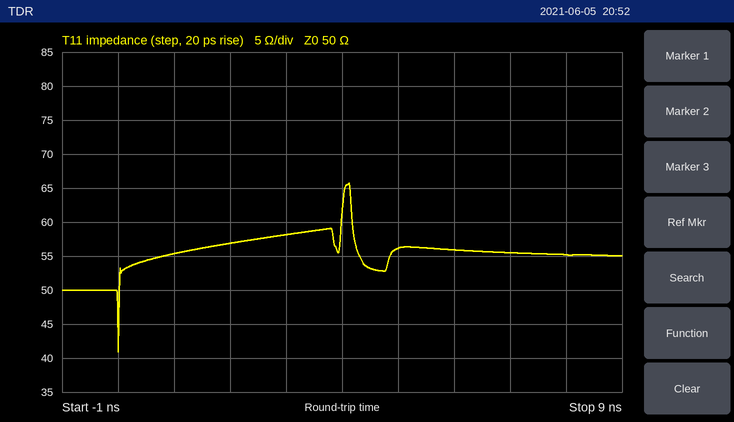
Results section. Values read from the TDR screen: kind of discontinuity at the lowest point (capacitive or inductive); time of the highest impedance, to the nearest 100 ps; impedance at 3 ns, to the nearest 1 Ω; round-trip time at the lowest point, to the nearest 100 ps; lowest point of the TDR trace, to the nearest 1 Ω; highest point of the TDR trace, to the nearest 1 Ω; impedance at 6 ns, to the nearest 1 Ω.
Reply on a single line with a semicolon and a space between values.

capacitive; 4.1 ns; 58 Ω; 0.0 ns; 41 Ω; 66 Ω; 56 Ω
